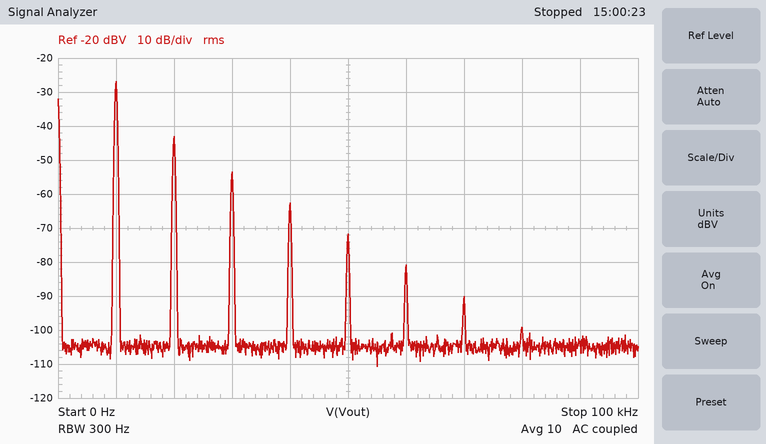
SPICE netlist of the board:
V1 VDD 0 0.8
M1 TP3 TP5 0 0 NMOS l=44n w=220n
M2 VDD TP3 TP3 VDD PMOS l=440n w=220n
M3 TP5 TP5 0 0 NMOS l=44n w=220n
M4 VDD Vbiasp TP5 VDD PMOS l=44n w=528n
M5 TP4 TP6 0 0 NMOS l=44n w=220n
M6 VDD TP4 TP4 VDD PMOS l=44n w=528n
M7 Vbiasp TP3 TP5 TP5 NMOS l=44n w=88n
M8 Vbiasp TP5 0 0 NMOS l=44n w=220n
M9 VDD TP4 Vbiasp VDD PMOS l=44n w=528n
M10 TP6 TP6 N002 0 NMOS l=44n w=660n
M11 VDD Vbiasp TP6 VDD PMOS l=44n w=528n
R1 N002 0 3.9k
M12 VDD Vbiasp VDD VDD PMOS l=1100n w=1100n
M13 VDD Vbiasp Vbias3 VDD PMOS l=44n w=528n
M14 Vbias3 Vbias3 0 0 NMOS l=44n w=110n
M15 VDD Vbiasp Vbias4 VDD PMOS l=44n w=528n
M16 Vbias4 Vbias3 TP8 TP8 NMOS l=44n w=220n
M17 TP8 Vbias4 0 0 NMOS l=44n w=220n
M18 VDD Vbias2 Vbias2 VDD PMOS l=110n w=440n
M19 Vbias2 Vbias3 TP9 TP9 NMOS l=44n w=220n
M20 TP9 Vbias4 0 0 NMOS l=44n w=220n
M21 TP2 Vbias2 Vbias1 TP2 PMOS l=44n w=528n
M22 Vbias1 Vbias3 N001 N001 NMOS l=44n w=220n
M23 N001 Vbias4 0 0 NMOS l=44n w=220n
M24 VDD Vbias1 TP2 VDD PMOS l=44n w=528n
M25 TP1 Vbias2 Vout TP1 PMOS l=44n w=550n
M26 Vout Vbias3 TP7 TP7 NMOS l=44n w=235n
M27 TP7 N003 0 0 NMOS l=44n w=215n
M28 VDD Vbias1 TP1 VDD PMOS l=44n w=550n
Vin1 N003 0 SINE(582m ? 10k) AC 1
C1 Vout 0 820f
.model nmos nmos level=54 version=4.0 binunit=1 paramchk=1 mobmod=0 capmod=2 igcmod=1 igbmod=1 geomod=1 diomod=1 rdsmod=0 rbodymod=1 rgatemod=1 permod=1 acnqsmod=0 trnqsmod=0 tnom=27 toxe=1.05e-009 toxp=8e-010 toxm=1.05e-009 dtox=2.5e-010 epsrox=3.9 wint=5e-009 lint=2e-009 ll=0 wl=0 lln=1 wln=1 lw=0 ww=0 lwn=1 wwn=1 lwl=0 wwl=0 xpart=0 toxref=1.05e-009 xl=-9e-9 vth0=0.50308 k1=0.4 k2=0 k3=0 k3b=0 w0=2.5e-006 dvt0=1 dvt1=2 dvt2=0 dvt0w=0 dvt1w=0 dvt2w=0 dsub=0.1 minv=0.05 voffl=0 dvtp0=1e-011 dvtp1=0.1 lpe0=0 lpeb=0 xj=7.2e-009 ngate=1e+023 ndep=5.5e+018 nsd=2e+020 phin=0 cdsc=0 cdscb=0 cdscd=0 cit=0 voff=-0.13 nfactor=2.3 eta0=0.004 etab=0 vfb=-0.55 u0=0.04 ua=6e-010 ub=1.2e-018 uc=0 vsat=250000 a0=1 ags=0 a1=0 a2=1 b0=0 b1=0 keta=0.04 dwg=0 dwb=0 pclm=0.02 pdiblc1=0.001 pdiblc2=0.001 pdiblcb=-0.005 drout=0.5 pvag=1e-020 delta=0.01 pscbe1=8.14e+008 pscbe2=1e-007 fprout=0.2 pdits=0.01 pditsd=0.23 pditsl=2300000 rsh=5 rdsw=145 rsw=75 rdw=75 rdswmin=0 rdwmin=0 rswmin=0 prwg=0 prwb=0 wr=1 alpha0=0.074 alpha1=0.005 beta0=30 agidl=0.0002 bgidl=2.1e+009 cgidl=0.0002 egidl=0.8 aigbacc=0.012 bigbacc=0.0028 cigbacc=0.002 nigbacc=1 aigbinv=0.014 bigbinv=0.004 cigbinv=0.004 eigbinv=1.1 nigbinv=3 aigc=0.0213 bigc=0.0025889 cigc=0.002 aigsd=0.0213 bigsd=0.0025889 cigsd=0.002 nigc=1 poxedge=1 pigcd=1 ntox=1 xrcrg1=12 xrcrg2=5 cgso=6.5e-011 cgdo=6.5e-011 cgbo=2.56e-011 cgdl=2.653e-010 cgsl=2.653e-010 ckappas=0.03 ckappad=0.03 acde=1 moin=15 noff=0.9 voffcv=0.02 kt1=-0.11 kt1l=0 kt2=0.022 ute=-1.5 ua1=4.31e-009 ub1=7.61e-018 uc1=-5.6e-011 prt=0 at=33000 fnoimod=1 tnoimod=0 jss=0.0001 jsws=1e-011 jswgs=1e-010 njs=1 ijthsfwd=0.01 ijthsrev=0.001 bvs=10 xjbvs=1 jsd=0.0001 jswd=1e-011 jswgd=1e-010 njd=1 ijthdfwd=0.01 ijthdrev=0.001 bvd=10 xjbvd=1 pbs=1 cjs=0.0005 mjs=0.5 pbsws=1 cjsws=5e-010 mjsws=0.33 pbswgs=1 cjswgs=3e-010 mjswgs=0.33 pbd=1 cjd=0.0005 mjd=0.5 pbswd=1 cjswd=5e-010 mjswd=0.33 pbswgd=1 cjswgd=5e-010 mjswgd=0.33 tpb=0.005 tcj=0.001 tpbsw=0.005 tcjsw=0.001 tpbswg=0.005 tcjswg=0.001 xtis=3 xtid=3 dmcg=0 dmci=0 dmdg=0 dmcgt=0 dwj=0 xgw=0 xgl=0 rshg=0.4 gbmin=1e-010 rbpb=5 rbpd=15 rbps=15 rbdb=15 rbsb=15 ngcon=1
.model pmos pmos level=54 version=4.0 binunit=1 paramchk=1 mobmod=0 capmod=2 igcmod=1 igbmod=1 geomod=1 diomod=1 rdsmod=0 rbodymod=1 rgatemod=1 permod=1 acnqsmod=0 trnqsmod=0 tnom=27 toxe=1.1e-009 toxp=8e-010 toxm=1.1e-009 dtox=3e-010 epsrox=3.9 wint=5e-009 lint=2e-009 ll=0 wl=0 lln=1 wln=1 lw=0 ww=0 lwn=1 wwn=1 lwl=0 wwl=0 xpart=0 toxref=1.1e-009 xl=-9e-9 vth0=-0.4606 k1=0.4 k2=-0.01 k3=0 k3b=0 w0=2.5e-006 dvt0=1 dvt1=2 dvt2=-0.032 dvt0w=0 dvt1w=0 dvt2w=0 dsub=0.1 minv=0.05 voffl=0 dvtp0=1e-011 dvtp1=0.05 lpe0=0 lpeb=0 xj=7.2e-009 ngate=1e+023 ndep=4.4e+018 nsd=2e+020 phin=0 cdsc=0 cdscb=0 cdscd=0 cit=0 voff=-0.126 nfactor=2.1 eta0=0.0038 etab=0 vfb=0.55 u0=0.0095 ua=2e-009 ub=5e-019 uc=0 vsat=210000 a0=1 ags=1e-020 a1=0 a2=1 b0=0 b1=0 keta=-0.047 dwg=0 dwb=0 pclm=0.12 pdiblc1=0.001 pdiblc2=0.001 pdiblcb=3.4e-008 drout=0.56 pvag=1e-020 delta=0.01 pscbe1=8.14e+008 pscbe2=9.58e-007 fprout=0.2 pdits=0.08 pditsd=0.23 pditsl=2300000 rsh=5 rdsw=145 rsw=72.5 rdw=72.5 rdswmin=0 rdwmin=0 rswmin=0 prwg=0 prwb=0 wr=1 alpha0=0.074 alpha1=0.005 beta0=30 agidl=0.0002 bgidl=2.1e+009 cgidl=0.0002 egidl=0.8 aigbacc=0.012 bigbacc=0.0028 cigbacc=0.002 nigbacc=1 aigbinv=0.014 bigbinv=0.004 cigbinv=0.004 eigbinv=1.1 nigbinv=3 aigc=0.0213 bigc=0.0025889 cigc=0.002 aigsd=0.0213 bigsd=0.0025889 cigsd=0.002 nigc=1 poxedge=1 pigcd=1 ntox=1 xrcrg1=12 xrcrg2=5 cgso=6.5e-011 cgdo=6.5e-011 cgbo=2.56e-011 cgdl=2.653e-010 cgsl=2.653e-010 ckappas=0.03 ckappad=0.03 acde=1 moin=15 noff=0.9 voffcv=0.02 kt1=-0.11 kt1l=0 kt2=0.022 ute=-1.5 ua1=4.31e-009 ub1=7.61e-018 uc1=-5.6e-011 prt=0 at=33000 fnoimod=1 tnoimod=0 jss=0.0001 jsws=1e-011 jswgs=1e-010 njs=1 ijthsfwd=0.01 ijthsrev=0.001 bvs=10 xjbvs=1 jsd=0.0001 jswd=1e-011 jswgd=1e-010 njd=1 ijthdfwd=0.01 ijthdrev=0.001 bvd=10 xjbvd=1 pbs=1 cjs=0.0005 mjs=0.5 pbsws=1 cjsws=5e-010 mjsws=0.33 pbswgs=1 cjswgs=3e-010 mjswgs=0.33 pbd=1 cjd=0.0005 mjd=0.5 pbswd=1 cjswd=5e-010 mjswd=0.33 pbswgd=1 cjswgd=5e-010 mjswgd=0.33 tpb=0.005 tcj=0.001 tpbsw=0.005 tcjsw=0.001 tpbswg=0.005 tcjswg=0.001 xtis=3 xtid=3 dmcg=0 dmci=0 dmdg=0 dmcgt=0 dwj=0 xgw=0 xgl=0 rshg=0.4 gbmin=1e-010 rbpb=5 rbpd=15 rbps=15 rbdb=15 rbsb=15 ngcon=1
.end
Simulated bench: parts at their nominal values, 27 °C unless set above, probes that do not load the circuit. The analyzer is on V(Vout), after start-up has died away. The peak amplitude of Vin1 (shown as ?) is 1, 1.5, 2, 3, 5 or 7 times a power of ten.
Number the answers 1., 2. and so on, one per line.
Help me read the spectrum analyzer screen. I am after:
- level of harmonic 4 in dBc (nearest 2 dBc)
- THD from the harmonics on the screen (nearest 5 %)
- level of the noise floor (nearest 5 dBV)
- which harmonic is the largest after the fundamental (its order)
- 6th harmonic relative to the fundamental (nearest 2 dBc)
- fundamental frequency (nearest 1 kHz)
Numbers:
1. -36 dBc
2. 15 %
3. -105 dBV
4. 2
5. -54 dBc
6. 10 kHz
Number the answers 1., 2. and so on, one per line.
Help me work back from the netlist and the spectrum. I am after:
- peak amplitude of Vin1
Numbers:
1. 20 mV
